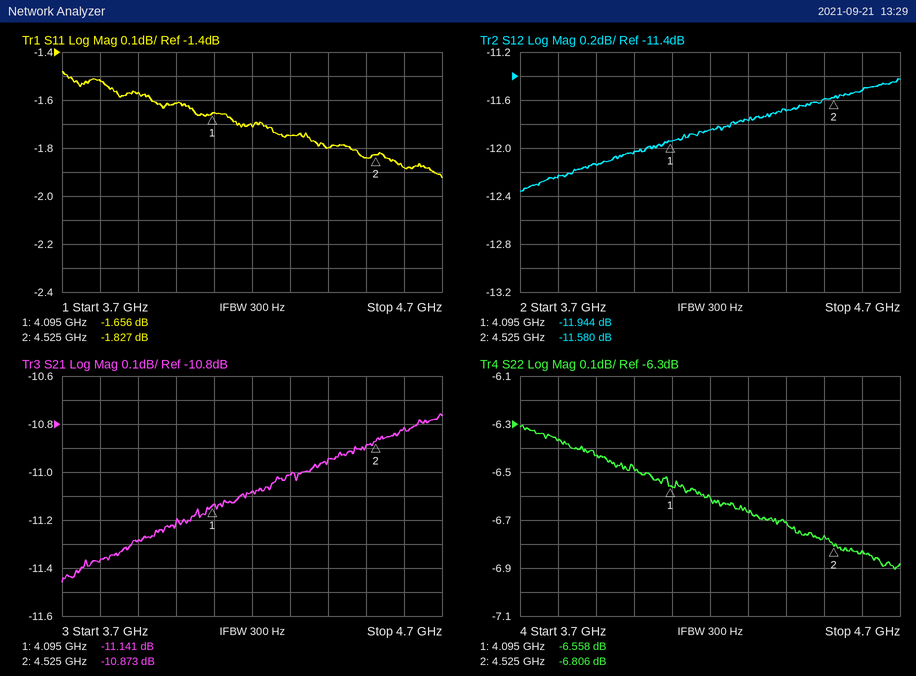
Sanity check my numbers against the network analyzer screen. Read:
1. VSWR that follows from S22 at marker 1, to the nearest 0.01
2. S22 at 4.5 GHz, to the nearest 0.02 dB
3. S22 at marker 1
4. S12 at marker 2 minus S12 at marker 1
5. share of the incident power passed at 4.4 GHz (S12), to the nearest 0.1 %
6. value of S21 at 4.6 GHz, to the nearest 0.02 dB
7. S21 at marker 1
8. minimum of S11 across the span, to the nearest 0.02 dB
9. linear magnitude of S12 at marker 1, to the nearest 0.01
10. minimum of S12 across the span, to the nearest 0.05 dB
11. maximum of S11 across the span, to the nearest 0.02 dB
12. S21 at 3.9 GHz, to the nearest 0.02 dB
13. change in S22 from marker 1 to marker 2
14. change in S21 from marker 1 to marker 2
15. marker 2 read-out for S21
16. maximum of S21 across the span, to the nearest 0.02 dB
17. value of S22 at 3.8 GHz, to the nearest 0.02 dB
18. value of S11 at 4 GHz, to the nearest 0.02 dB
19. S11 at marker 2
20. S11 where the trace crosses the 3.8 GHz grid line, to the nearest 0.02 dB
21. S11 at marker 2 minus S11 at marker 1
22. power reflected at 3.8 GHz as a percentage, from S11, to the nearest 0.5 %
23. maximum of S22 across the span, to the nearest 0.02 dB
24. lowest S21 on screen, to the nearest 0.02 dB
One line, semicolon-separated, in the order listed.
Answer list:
2.77; -6.76 dB; -6.558 dB; 0.364 dB; 6.8 %; -10.82 dB; -11.141 dB; -1.92 dB; 0.25; -12.35 dB; -1.48 dB; -11.28 dB; -0.248 dB; 0.268 dB; -10.873 dB; -10.76 dB; -6.36 dB; -1.62 dB; -1.827 dB; -1.52 dB; -0.171 dB; 70.5 %; -6.30 dB; -11.46 dB
